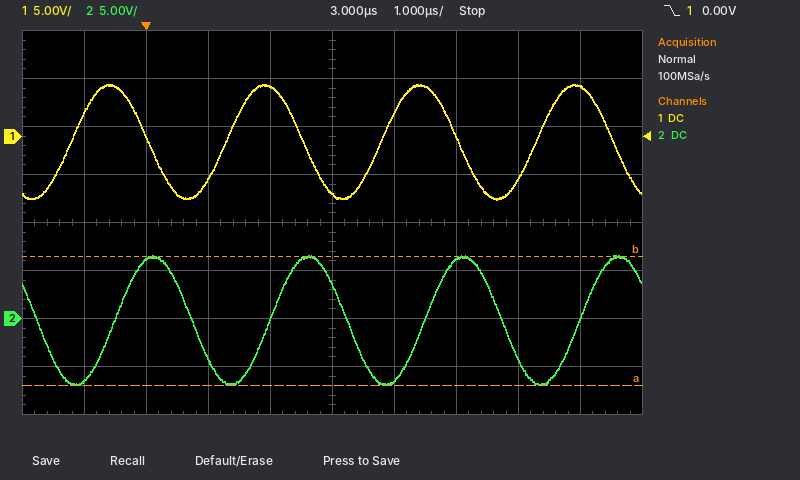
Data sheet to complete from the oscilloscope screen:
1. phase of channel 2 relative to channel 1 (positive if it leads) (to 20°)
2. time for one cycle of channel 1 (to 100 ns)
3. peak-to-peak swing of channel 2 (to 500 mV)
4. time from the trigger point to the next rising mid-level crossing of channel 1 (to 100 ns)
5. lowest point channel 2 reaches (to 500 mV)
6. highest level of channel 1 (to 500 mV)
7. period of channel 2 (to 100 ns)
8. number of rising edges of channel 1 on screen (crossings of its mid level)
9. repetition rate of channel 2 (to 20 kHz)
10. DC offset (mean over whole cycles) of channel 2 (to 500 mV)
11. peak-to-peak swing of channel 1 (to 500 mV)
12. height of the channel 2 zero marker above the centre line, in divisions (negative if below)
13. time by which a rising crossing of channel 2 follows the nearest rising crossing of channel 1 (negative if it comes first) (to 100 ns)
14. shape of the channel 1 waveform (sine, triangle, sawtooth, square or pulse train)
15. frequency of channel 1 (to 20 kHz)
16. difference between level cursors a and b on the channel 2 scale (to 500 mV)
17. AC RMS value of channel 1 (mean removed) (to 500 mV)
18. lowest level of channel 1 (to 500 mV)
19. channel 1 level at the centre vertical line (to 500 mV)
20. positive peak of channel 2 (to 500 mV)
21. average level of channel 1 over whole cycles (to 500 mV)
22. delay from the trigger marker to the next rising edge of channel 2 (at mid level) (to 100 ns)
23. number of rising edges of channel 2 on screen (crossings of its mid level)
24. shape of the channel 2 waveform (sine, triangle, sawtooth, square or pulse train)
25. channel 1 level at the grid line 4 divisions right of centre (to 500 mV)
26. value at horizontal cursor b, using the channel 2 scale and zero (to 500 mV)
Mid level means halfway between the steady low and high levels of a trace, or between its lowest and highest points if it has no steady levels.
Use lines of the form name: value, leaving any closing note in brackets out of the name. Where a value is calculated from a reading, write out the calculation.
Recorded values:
phase of channel 2 relative to channel 1 (positive if it leads): −360° × (+700 ns) / 2.5 µs ≈ -101°, so -100° to the nearest 20°
time for one cycle of channel 1: 2.5 µs
peak-to-peak swing of channel 2: 6.5 V − (-7.0 V) = 13.5 V
time from the trigger point to the next rising mid-level crossing of channel 1: 1.3 µs
lowest point channel 2 reaches: -7.0 V
highest level of channel 1: 5.5 V
period of channel 2: 2.5 µs
number of rising edges of channel 1 on screen: 4
repetition rate of channel 2: 1 / 2.5 µs ≈ 400 kHz
DC offset (mean over whole cycles) of channel 2: (6.5 V + (-7.0 V)) / 2 ≈ 0.0 V
peak-to-peak swing of channel 1: 5.5 V − (-6.5 V) = 12.0 V
height of the channel 2 zero marker above the centre line, in divisions: -2.0 div
time by which a rising crossing of channel 2 follows the nearest rising crossing of channel 1 (negative if it comes first): +700 ns
shape of the channel 1 waveform: sine
frequency of channel 1: 1 / 2.5 µs ≈ 400 kHz
difference between level cursors a and b on the channel 2 scale: 13.5 V
AC RMS value of channel 1 (mean removed): 12.0 V / (2√2) ≈ 4.24 V, so 4.0 V to the nearest 500 mV
lowest level of channel 1: -6.5 V
channel 1 level at the centre vertical line: -6.0 V
positive peak of channel 2: 6.5 V
average level of channel 1 over whole cycles: (5.5 V + (-6.5 V)) / 2 ≈ -500 mV
delay from the trigger marker to the next rising edge of channel 2 (at mid level): 2.0 µs
number of rising edges of channel 2 on screen: 4
shape of the channel 2 waveform: sine
channel 1 level at the grid line 4 divisions right of centre: 5.0 V
value at horizontal cursor b, using the channel 2 scale and zero: 6.5 V
